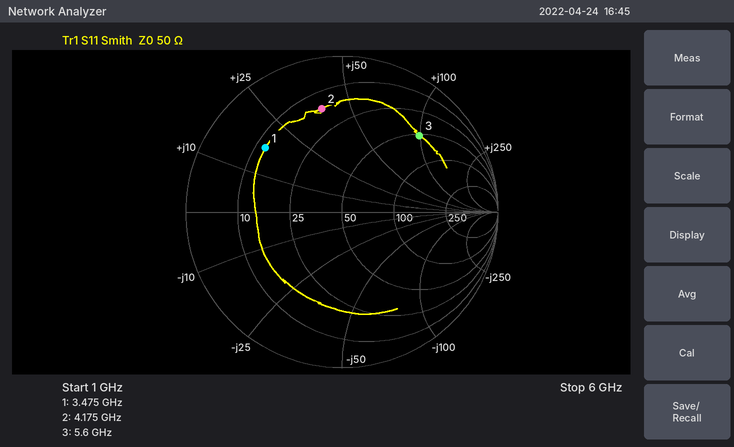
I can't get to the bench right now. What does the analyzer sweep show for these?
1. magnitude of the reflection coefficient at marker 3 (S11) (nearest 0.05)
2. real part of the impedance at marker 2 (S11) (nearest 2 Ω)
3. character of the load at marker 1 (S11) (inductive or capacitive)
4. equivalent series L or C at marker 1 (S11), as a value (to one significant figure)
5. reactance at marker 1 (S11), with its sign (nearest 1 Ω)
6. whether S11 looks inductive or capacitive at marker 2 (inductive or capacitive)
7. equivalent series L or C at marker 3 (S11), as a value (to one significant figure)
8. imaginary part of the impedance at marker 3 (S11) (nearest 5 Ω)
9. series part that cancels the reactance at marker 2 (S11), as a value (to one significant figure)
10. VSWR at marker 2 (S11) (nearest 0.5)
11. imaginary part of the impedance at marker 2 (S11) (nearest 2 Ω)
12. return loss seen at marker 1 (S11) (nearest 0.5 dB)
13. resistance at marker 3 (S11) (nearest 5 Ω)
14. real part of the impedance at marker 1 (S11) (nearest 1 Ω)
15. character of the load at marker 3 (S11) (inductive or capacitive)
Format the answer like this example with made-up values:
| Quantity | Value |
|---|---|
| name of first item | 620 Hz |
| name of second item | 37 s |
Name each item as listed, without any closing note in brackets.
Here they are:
| Quantity | Value |
|---|---|
| magnitude of the reflection coefficient at marker 3 (S11) | 0.70 |
| real part of the impedance at marker 2 (S11) | 16 Ω |
| character of the load at marker 1 (S11) | inductive |
| equivalent series L or C at marker 1 (S11), as a value | 800 pH |
| reactance at marker 1 (S11), with its sign | +17 Ω |
| whether S11 looks inductive or capacitive at marker 2 | inductive |
| equivalent series L or C at marker 3 (S11), as a value | 3 nH |
| imaginary part of the impedance at marker 3 (S11) | +100 Ω |
| series part that cancels the reactance at marker 2 (S11), as a value | 1.0 pF |
| VSWR at marker 2 (S11) | 5.0 |
| imaginary part of the impedance at marker 2 (S11) | +38 Ω |
| return loss seen at marker 1 (S11) | 4.0 dB |
| resistance at marker 3 (S11) | 50 Ω |
| real part of the impedance at marker 1 (S11) | 12 Ω |
| character of the load at marker 3 (S11) | inductive |
